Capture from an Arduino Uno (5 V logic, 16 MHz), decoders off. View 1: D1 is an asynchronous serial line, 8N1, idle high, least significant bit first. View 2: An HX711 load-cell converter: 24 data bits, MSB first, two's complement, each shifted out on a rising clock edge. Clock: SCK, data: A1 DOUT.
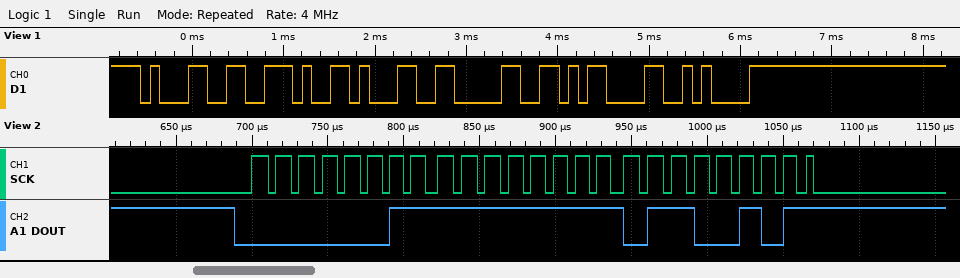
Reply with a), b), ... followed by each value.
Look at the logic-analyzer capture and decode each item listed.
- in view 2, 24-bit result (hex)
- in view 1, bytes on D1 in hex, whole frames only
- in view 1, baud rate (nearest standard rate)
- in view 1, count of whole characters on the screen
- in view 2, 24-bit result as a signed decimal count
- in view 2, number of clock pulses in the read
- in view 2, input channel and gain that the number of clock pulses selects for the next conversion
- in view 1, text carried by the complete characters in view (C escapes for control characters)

a) 0x03FF65
b) 31 2E 31 30 0D 0A
c) 9600 baud
d) 6
e) 261989
f) 25
g) channel A, gain 128
h) "1.10\r\n"
